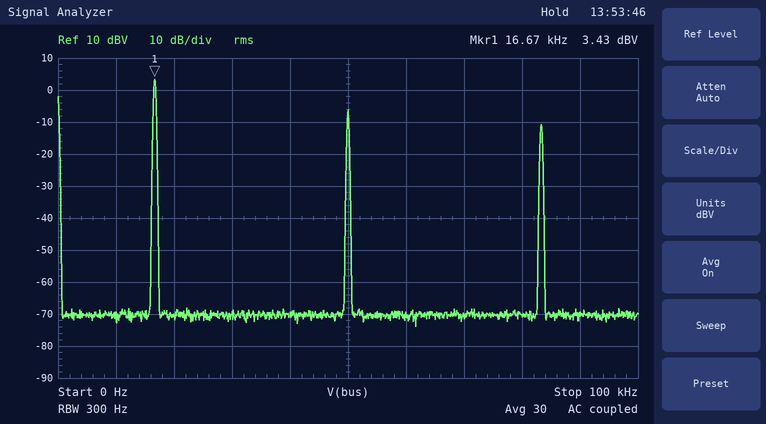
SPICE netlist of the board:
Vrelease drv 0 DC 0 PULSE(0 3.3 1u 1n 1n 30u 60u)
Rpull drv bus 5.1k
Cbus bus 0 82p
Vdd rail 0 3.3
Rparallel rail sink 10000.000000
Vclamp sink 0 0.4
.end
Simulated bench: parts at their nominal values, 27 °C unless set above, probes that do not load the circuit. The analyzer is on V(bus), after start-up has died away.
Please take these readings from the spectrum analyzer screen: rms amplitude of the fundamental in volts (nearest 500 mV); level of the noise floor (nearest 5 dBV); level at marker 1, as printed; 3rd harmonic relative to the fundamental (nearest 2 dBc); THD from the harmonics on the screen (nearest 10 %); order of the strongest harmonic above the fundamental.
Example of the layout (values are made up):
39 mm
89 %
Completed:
1.5 V
-70 dBV
3.43 dBV
-10 dBc
40 %
3
